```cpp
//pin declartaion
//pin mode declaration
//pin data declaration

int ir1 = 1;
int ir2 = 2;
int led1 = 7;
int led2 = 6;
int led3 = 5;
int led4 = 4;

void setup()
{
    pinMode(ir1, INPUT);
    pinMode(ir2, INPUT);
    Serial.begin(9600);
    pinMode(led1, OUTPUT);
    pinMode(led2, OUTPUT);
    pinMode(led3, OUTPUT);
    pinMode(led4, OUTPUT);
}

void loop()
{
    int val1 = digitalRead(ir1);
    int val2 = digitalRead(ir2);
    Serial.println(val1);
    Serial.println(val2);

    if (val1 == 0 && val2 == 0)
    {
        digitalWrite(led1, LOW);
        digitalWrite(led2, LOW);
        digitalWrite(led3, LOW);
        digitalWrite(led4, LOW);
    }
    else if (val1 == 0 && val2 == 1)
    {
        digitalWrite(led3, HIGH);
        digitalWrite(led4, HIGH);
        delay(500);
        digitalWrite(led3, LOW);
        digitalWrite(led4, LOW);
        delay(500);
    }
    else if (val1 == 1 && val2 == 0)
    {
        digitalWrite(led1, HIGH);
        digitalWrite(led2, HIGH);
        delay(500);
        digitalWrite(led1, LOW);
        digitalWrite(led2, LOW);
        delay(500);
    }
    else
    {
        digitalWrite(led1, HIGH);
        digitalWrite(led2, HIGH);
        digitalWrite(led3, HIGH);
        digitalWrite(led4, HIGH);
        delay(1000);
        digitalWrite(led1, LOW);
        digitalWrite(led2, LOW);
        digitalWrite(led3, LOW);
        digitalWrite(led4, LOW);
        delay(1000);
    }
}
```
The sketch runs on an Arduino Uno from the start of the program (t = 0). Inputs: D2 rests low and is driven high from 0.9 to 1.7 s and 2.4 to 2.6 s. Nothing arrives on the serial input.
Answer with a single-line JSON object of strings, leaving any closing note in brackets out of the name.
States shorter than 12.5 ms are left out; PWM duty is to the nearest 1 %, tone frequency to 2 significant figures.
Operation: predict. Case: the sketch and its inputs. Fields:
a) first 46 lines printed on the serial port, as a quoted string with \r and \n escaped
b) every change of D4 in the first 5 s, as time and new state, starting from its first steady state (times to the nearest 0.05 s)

{"first 46 lines printed on the serial port, as a quoted string with \\r and \\n escaped": "\"0\\r\\n0\\r\\n0\\r\\n0\\r\\n0\\r\\n0\\r\\n0\\r\\n0\\r\\n0\\r\\n0\\r\\n0\\r\\n0\\r\\n0\\r\\n0\\r\\n0\\r\\n0\\r\\n0\\r\\n0\\r\\n0\\r\\n0\\r\\n0\\r\\n0\\r\\n0\\r\\n0\\r\\n0\\r\\n0\\r\\n0\\r\\n0\\r\\n0\\r\\n0\\r\\n0\\r\\n0\\r\\n0\\r\\n0\\r\\n0\\r\\n0\\r\\n0\\r\\n0\\r\\n0\\r\\n0\\r\\n0\\r\\n0\\r\\n0\\r\\n0\\r\\n0\\r\\n0\\r\\n\"", "every change of D4 in the first 5 s, as time and new state, starting from its first steady state": "0 s low; 0.9 s high; 1.4 s low; 2.4 s high; 2.9 s low"}
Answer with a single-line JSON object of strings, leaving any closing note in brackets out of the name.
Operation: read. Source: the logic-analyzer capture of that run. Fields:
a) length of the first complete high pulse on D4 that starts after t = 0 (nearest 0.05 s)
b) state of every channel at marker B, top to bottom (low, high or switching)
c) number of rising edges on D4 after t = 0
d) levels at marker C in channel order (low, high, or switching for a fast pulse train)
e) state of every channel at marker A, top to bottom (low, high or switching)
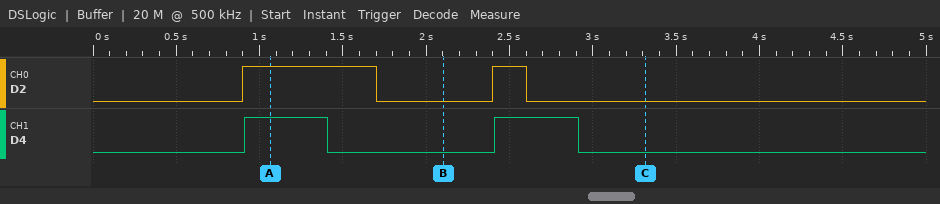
{"length of the first complete high pulse on D4 that starts after t = 0": "0.50 s", "state of every channel at marker B, top to bottom": "D2 low, D4 low", "number of rising edges on D4 after t = 0": "2", "levels at marker C in channel order": "D2 low, D4 low", "state of every channel at marker A, top to bottom": "D2 high, D4 high"}
